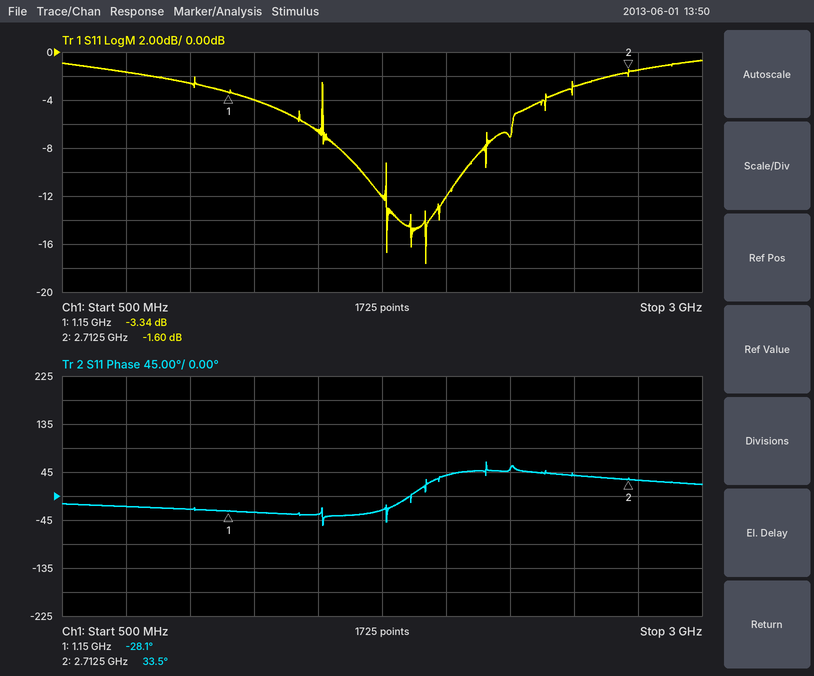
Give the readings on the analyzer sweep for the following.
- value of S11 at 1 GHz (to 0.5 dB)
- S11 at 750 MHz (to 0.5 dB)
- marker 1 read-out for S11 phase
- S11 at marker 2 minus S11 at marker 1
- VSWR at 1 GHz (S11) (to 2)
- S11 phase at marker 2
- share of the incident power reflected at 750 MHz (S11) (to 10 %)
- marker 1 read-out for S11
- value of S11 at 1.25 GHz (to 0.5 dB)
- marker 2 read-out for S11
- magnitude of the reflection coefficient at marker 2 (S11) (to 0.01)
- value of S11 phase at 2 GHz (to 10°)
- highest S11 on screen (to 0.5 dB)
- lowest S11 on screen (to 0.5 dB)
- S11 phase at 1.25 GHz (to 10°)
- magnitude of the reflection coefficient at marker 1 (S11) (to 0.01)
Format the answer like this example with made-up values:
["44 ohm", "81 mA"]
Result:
["-2.5 dB", "-1.5 dB", "-28.1°", "1.74 dB", "6", "33.5°", "70 %", "-3.34 dB", "-4.0 dB", "-1.60 dB", "0.83", "40°", "-0.5 dB", "-17.5 dB", "-30°", "0.68"]
